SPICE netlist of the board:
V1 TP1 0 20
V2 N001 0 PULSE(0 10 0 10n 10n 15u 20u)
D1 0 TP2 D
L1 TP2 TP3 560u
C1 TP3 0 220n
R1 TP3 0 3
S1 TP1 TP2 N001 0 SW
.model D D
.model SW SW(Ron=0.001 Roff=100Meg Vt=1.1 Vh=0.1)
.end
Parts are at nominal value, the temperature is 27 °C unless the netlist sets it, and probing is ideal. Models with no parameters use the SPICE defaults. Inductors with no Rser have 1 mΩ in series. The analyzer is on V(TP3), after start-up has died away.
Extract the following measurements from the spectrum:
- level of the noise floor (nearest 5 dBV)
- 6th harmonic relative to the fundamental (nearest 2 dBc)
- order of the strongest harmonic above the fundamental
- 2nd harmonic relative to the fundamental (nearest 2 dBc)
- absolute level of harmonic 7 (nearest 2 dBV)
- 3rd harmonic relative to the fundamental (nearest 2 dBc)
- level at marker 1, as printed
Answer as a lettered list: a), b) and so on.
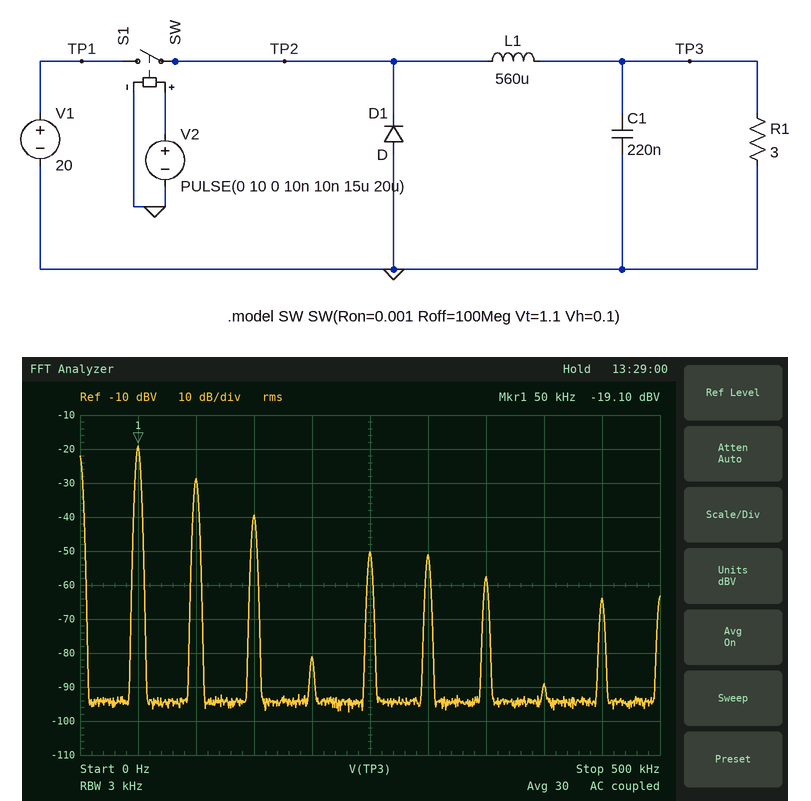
a) -95 dBV
b) -32 dBc
c) 2
d) -10 dBc
e) -58 dBV
f) -20 dBc
g) -19.10 dBV
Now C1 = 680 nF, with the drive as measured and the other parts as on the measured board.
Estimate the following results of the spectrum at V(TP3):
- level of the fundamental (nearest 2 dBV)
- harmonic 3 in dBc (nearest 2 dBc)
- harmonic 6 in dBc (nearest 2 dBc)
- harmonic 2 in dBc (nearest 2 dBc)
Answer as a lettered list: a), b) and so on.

a) -20 dBV
b) -24 dBc
c) -38 dBc
d) -12 dBc
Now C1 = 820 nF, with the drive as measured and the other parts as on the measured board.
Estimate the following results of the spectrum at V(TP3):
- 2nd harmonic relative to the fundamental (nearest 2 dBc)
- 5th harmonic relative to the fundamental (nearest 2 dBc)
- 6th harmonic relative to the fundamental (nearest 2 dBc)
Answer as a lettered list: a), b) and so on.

a) -12 dBc
b) -38 dBc
c) -40 dBc
